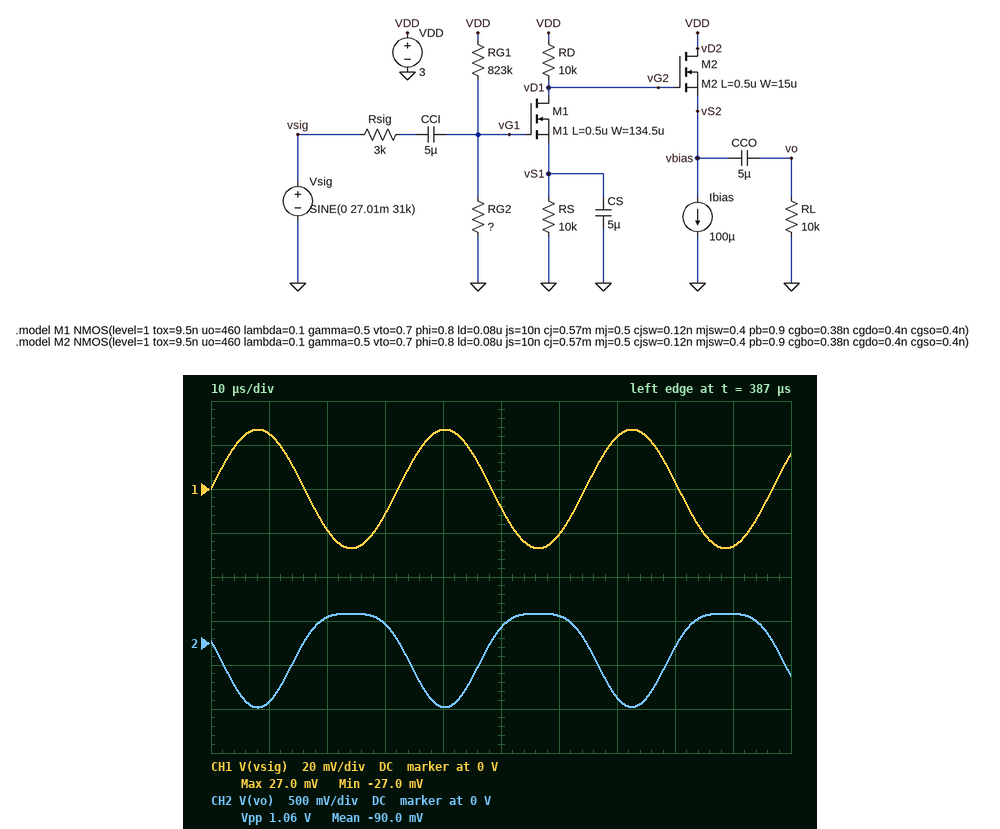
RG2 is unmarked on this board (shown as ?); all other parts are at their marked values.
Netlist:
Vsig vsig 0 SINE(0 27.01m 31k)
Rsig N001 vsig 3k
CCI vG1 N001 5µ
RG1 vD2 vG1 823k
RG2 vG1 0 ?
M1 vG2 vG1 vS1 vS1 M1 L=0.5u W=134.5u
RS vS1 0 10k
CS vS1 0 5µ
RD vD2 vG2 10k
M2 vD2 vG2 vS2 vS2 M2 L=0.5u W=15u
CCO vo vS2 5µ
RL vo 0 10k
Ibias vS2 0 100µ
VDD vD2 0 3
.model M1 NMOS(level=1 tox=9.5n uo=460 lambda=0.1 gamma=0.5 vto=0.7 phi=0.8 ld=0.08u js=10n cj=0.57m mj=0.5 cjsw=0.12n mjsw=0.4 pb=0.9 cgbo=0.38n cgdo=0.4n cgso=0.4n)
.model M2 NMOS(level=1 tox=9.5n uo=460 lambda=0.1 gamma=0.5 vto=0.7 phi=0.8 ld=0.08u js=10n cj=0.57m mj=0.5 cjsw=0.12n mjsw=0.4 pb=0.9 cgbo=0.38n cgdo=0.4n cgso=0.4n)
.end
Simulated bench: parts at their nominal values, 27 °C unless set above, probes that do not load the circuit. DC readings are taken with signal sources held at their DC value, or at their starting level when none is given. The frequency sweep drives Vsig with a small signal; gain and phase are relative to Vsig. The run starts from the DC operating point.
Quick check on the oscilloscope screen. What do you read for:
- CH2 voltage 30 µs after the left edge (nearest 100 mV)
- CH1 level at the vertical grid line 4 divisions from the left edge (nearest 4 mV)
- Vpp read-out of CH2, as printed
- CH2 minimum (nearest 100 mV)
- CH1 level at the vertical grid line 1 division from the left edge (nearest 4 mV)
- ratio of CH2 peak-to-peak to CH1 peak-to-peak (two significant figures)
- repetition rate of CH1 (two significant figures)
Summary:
200 mV
28 mV
1.06 V
-700 mV
24 mV
20
31 kHz
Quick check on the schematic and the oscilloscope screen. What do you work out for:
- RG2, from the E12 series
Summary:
470 kΩ
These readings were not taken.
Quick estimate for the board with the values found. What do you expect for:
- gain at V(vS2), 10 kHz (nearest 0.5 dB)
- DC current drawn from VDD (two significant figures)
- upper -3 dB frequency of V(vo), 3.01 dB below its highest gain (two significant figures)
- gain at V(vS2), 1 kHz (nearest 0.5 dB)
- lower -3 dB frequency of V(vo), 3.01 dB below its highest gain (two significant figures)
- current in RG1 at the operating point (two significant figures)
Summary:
26.5 dB
140 µA
32 MHz
26.5 dB
78 Hz
2.3 µA
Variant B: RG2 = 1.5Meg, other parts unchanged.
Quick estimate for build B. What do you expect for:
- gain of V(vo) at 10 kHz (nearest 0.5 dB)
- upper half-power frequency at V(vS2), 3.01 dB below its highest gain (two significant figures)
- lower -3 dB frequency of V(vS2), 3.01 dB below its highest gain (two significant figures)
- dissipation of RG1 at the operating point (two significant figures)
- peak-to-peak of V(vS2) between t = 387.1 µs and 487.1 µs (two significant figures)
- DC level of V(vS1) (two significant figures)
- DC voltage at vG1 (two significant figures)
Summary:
30.5 dB
23 MHz
120 Hz
1.4 µW
1.3 V
1.2 V
1.9 V
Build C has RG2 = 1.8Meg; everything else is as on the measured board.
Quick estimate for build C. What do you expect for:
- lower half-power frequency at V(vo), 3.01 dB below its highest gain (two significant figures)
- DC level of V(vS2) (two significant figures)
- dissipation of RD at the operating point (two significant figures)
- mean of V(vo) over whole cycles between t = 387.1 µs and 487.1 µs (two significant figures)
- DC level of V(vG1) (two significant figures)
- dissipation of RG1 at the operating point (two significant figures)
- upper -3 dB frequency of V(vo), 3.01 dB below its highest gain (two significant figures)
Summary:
120 Hz
850 mV
170 µW
98 mV
2.1 V
1.1 µW
22 MHz
